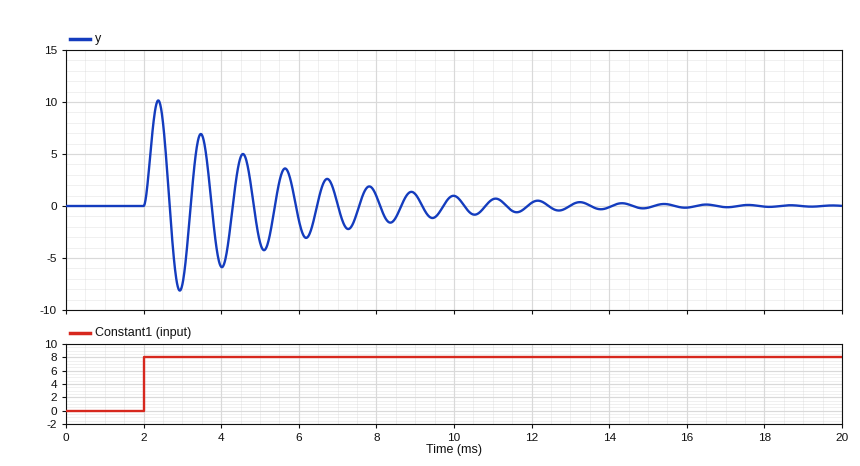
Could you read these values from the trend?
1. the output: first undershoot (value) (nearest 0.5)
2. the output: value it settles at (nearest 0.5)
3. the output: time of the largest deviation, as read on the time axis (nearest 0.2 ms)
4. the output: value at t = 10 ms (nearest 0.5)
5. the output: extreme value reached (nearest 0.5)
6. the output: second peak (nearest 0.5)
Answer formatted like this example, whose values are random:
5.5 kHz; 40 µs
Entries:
-8.0; 0.0; 2.4 ms; 1.0; 10.0; 7.0
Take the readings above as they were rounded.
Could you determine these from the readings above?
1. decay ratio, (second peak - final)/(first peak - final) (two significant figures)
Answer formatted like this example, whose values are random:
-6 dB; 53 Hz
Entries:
0.70
